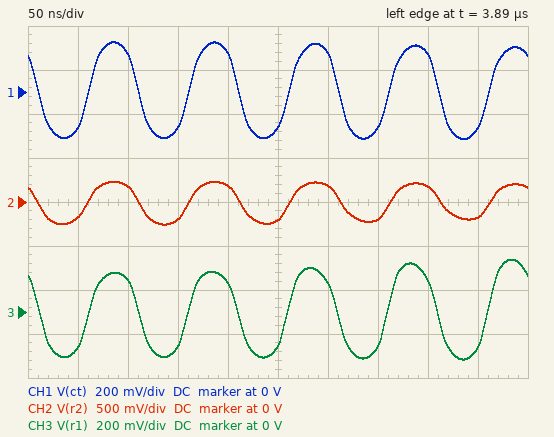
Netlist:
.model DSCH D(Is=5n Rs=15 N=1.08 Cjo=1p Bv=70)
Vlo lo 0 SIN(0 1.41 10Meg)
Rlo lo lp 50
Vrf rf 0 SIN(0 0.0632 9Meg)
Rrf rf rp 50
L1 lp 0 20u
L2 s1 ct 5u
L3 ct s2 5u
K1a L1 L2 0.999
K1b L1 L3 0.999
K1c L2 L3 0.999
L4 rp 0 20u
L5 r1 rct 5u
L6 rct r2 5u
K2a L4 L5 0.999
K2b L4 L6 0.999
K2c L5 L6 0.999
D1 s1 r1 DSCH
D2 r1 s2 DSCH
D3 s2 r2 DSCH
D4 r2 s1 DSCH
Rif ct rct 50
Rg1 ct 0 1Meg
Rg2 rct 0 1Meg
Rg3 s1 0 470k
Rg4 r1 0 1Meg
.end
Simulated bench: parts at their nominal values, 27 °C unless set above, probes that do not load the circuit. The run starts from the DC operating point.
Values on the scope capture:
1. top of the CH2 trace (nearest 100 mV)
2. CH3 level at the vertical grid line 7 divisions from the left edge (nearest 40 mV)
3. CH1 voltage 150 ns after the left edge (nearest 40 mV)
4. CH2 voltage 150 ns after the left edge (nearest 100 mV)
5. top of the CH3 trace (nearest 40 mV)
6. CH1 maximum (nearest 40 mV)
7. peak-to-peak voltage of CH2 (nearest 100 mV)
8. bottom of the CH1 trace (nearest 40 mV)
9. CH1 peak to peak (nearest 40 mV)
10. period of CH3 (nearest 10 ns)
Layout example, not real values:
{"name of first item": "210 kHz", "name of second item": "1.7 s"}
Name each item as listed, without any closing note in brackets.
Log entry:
{"top of the CH2 trace": "200 mV", "CH3 level at the vertical grid line 7 divisions from the left edge": "-160 mV", "CH1 voltage 150 ns after the left edge": "-160 mV", "CH2 voltage 150 ns after the left edge": "-200 mV", "top of the CH3 trace": "240 mV", "CH1 maximum": "240 mV", "peak-to-peak voltage of CH2": "500 mV", "bottom of the CH1 trace": "-200 mV", "CH1 peak to peak": "440 mV", "period of CH3": "100 ns"}
